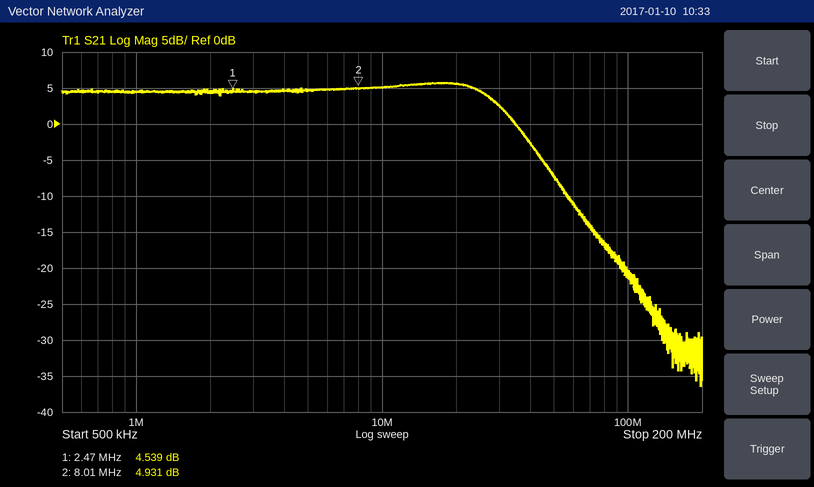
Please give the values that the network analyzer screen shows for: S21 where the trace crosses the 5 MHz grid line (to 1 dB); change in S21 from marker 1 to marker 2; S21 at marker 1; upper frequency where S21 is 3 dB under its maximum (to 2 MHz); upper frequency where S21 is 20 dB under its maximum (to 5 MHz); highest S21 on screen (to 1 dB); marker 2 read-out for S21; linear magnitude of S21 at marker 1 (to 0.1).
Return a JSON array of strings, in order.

["5 dB", "0.392 dB", "4.539 dB", "30 MHz", "70 MHz", "6 dB", "4.931 dB", "1.7"]
